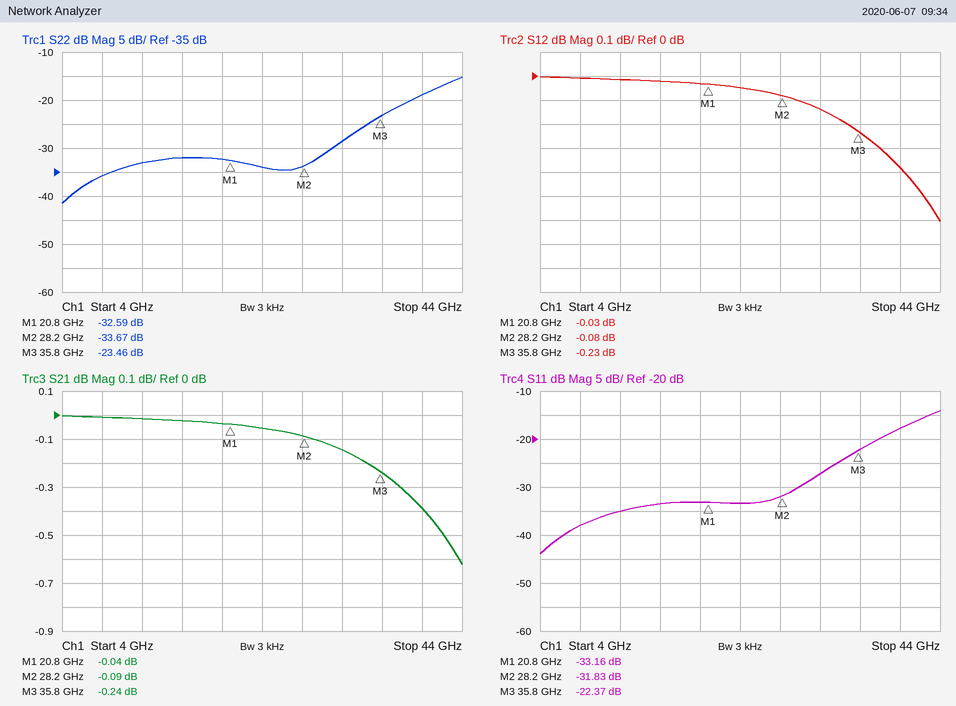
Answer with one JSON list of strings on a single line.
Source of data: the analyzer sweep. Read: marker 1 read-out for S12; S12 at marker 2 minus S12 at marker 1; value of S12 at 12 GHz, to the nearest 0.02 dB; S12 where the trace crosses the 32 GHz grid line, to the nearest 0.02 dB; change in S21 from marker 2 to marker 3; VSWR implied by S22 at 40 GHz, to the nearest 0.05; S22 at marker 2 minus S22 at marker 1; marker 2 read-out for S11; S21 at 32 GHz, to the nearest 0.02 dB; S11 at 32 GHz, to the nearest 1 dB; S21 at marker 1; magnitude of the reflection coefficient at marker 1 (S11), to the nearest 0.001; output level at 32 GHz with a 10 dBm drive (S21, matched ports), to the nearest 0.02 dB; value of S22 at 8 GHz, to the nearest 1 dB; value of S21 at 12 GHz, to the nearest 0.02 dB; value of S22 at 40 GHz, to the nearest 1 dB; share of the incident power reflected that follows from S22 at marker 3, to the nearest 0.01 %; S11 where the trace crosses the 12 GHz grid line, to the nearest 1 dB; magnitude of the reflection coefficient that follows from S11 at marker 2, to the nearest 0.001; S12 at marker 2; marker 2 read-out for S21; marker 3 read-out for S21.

["-0.03 dB", "-0.05 dB", "-0.02 dB", "-0.14 dB", "-0.15 dB", "1.25", "-1.08 dB", "-31.83 dB", "-0.14 dB", "-27 dB", "-0.04 dB", "0.022", "9.86 dBm", "-36 dB", "-0.02 dB", "-19 dB", "0.45 %", "-35 dB", "0.026", "-0.08 dB", "-0.09 dB", "-0.24 dB"]
